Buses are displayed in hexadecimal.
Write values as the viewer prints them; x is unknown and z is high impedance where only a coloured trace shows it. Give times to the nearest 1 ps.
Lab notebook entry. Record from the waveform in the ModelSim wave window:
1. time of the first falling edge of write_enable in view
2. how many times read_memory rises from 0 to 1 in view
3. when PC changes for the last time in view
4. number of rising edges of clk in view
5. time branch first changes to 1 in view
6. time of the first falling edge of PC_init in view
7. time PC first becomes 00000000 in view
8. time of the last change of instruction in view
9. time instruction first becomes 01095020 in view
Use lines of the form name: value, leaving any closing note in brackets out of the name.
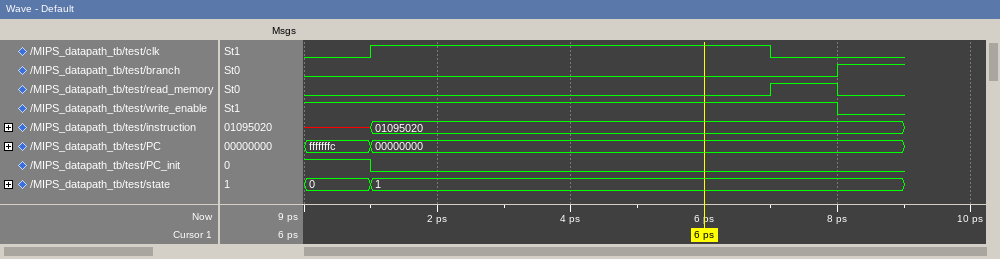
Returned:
time of the first falling edge of write_enable in view: 8 ps
how many times read_memory rises from 0 to 1 in view: 1
when PC changes for the last time in view: 1 ps
number of rising edges of clk in view: 1
time branch first changes to 1 in view: 8 ps
time of the first falling edge of PC_init in view: 1 ps
time PC first becomes 00000000 in view: 1 ps
time of the last change of instruction in view: 1 ps
time instruction first becomes 01095020 in view: 1 ps
